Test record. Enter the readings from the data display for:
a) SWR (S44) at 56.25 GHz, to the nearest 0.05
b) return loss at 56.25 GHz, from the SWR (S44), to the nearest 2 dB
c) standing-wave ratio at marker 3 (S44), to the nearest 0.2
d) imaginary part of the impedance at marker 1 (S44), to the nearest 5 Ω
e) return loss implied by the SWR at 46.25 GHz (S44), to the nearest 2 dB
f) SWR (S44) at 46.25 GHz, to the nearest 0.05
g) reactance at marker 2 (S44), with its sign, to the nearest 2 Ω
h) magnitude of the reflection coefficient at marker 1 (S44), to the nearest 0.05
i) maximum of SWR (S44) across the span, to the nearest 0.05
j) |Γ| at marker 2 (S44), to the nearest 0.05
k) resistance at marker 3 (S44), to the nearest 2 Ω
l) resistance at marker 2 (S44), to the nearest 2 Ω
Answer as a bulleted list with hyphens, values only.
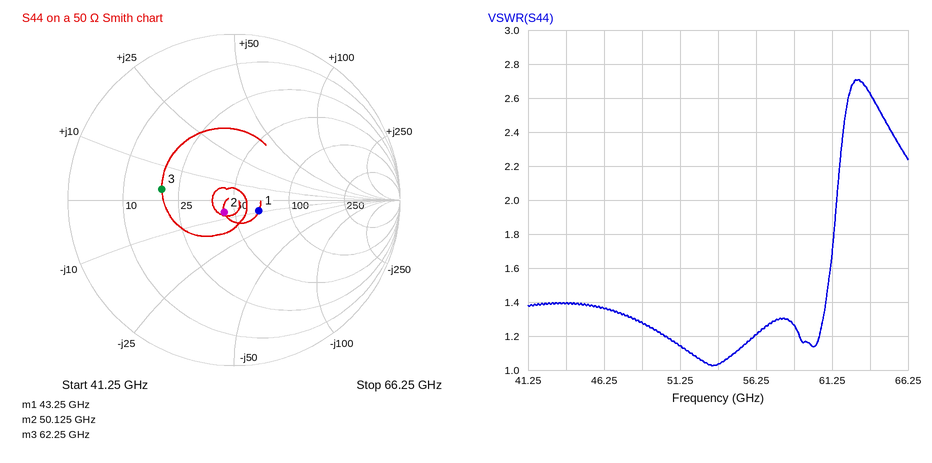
- 1.20
- 20 dB
- 2.6
- -10 Ω
- 16 dB
- 1.35
- -6 Ω
- 0.15
- 2.70
- 0.10
- 20 Ω
- 44 Ω
